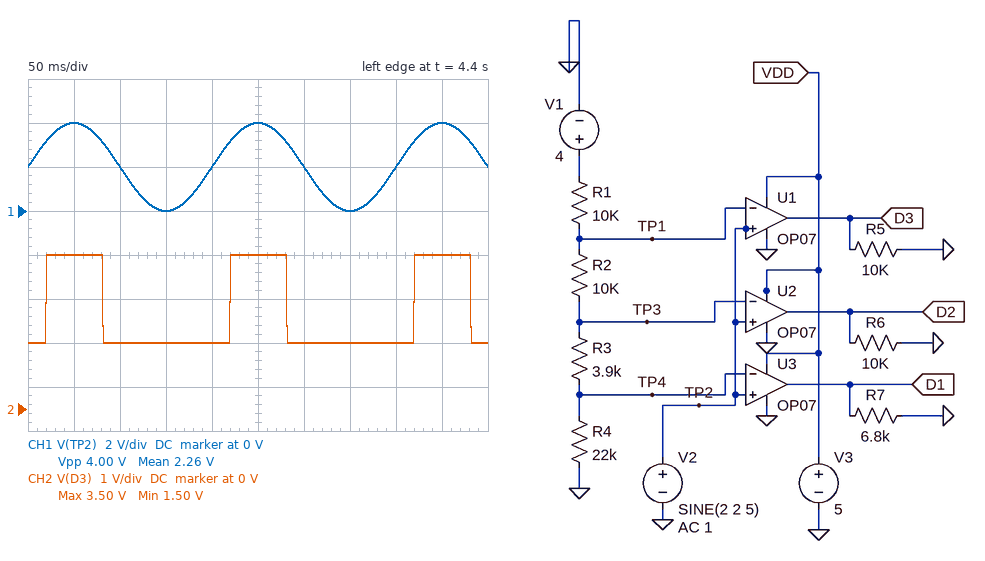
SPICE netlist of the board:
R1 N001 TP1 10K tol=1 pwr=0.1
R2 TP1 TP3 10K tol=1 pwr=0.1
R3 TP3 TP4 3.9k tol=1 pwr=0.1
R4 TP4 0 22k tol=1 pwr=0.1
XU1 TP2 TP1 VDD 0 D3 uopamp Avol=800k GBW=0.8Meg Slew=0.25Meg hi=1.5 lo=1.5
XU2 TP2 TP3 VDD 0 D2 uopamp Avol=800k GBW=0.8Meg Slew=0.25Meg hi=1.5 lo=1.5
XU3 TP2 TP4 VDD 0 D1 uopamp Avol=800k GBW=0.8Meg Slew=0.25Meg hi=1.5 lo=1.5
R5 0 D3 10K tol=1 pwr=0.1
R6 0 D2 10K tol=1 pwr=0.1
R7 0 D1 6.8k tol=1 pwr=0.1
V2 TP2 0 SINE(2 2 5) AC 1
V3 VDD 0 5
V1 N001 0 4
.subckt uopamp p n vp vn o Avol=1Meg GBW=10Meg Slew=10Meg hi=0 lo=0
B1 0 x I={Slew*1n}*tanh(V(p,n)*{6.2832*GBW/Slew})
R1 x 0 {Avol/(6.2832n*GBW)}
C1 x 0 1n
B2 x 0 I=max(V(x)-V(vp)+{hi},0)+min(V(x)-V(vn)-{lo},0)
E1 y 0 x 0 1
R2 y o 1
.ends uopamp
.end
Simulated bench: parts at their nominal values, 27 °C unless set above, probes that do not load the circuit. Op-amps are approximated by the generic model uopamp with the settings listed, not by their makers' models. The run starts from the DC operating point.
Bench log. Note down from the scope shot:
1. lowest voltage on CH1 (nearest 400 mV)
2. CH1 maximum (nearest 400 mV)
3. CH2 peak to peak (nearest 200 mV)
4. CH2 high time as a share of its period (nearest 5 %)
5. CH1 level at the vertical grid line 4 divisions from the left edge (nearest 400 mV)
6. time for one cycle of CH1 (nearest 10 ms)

0 V
4.0 V
2.0 V
30 %
2.0 V
200 ms
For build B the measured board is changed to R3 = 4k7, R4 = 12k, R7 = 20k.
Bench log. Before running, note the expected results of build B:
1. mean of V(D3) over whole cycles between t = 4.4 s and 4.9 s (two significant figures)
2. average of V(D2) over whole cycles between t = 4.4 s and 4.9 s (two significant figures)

2.2 V
2.6 V
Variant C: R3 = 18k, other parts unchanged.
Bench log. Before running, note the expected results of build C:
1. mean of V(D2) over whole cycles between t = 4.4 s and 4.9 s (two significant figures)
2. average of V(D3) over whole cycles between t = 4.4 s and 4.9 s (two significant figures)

2.3 V
2.0 V
